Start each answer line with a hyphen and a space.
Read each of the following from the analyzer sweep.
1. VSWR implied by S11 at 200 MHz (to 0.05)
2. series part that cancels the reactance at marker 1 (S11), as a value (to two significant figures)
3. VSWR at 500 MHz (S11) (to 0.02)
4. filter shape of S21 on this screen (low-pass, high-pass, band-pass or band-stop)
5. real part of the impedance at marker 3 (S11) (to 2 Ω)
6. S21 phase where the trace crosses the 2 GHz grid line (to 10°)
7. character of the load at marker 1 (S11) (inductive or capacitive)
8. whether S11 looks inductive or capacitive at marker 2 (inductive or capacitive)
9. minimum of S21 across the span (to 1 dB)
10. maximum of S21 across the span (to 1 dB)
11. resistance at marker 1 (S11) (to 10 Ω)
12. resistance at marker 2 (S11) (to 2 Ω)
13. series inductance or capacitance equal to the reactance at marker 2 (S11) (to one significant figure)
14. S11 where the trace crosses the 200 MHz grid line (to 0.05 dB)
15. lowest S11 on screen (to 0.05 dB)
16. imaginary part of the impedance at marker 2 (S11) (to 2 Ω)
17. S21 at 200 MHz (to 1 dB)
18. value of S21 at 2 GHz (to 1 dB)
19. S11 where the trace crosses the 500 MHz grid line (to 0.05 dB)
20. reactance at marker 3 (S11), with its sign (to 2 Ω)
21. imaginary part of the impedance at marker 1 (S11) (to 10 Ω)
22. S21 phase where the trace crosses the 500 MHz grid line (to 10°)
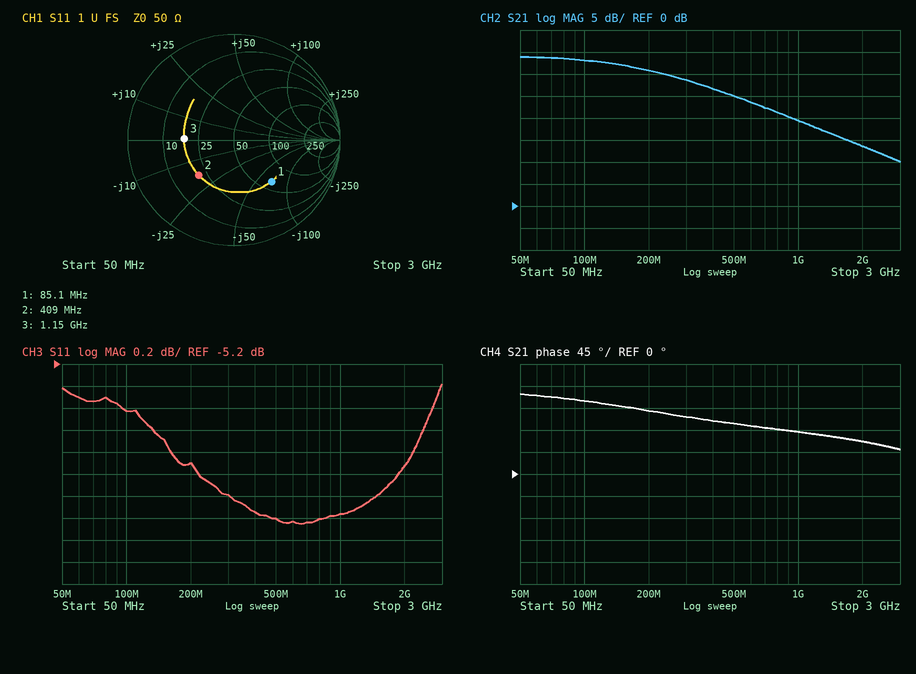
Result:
- 2.95
- 130 nH
- 2.76
- low-pass
- 18 Ω
- 70°
- capacitive
- capacitive
- 10 dB
- 34 dB
- 60 Ω
- 20 Ω
- 20 pF
- -6.10 dB
- -6.65 dB
- -18 Ω
- 31 dB
- 14 dB
- -6.60 dB
- 0 Ω
- -70 Ω
- 100°
